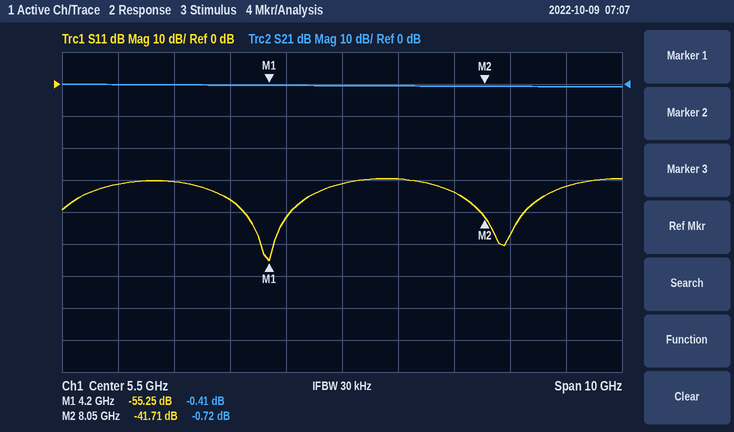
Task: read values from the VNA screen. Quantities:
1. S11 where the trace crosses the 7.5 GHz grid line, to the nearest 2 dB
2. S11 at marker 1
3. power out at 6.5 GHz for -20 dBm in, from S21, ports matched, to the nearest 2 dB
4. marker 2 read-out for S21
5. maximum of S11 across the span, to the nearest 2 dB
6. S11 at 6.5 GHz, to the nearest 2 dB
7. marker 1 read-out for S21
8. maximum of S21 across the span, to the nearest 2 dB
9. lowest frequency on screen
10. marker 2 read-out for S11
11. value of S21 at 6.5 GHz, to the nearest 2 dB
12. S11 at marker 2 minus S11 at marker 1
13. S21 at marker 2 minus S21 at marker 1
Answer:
-34 dB
-55.25 dB
-20 dBm
-0.72 dB
-30 dB
-30 dB
-0.41 dB
0 dB
500 MHz
-41.71 dB
0 dB
13.54 dB
-0.31 dB
